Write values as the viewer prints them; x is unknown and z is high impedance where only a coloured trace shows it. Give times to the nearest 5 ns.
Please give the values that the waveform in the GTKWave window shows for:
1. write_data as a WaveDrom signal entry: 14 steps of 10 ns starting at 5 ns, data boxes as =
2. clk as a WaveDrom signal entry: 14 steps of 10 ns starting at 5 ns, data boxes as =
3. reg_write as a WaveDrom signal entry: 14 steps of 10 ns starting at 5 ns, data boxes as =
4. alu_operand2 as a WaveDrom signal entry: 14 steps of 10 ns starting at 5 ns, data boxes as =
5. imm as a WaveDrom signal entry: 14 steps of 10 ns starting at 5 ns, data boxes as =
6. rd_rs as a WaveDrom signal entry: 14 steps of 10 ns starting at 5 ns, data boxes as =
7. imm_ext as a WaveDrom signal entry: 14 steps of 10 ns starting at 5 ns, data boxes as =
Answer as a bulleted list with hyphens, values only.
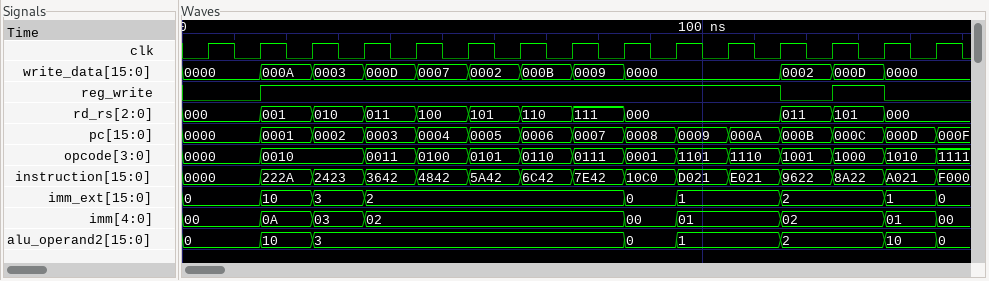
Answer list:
- {name: 'write_data', wave: '=========..===', data: '0000 000A 0003 000D 0007 0002 000B 0009 0000 0002 000D 0000'}
- {name: 'clk', wave: 'p.............'}
- {name: 'reg_write', wave: '01.........010'}
- {name: 'alu_operand2', wave: '===.....==.=.=', data: '0 10 3 0 1 2 10'}
- {name: 'imm', wave: '====....==.=.=', data: '00 0A 03 02 00 01 02 01'}
- {name: 'rd_rs', wave: '=========..===', data: '000 001 010 011 100 101 110 111 000 011 101 000'}
- {name: 'imm_ext', wave: '====....==.=.=', data: '0 10 3 2 0 1 2 1'}
